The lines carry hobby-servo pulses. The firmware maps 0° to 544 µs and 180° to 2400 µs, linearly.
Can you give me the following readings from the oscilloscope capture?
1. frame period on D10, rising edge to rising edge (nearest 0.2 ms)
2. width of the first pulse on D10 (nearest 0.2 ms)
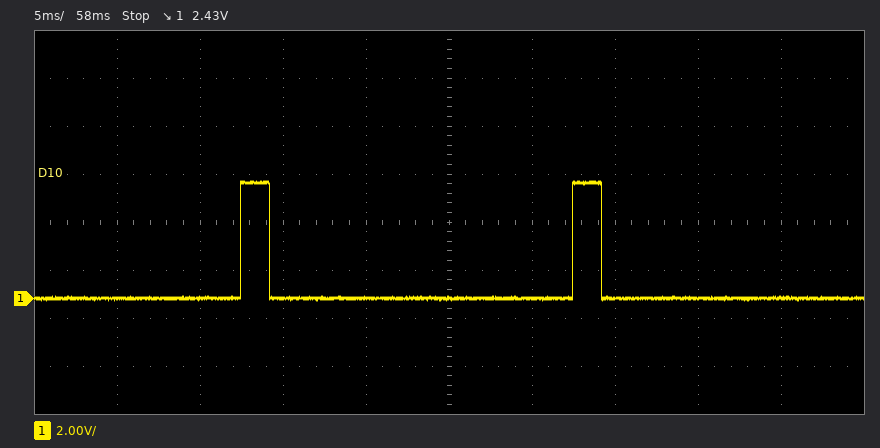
20.0 ms
1.8 ms
